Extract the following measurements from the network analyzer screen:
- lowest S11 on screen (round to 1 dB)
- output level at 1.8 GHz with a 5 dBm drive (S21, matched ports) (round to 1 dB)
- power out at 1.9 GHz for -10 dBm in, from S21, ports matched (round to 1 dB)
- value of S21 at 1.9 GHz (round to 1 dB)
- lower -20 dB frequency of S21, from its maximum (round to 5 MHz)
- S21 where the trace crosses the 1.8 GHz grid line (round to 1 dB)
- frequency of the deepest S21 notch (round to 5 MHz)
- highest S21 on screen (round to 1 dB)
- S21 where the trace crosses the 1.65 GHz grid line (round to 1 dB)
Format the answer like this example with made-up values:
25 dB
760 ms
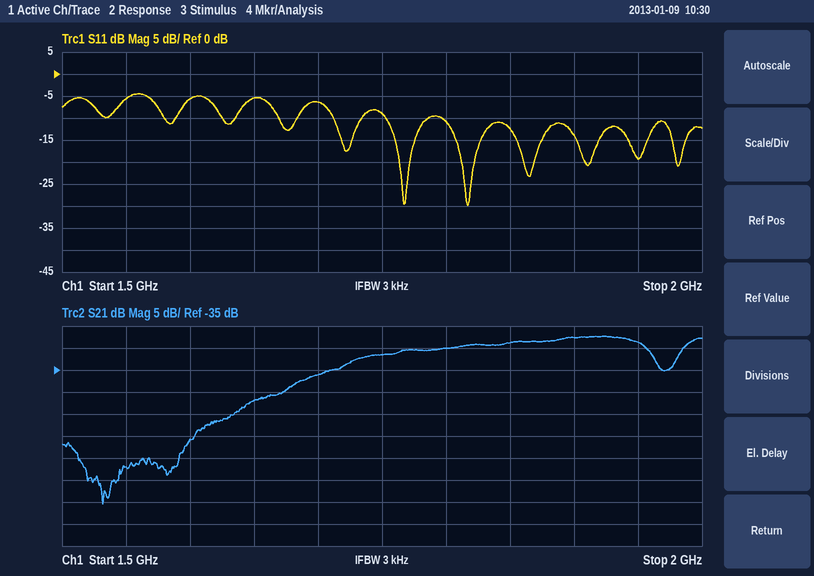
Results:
-30 dB
-25 dBm
-38 dBm
-28 dB
1.615 GHz
-30 dB
1.530 GHz
-27 dB
-42 dB
